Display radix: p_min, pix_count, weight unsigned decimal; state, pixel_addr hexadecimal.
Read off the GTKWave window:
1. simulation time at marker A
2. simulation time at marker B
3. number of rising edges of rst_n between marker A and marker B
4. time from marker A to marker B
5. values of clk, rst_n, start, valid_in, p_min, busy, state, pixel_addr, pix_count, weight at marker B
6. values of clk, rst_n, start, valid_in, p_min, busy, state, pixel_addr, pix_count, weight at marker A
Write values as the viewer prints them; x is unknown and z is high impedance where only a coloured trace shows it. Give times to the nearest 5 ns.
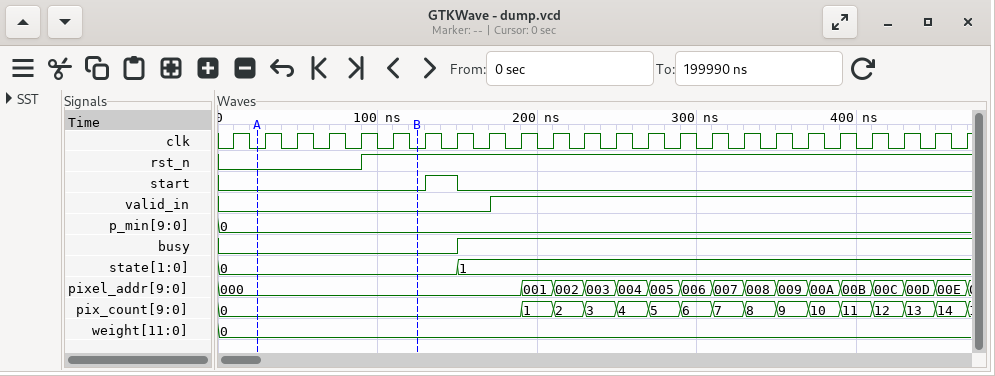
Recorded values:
25 ns
125 ns
1
100 ns
clk=0, rst_n=1, start=0, valid_in=0, p_min=0, busy=0, state=0, pixel_addr=000, pix_count=0, weight=0
clk=0, rst_n=0, start=0, valid_in=0, p_min=0, busy=0, state=0, pixel_addr=000, pix_count=0, weight=0
